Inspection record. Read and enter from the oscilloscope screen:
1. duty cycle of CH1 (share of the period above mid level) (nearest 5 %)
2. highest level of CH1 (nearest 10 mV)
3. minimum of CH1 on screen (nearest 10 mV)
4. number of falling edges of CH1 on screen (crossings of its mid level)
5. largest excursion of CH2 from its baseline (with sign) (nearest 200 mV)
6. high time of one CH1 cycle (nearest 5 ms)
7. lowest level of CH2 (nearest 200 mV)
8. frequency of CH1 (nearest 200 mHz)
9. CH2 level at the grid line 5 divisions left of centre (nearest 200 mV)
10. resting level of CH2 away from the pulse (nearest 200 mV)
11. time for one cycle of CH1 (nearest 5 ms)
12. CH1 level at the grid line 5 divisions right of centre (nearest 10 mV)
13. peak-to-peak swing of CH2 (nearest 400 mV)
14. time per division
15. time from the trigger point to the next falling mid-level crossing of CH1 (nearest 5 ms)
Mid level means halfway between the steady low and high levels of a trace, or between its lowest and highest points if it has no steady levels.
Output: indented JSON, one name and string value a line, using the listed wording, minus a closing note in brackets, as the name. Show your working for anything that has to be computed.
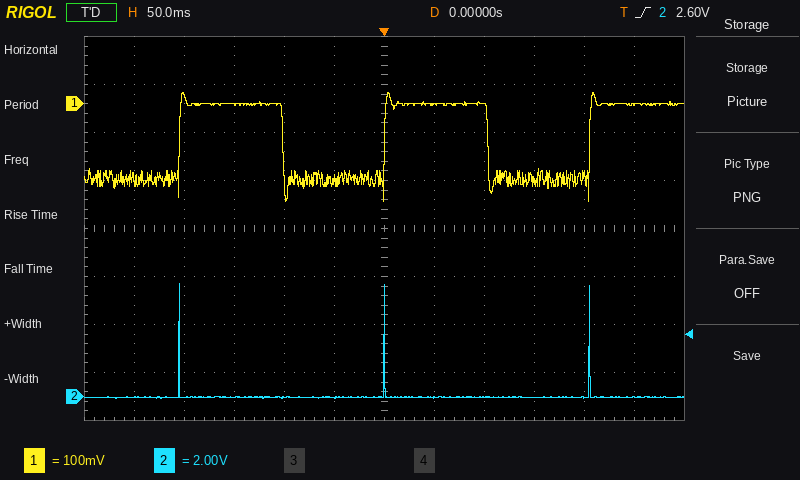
{
  "duty cycle of CH1 (share of the period above mid level)": "105 ms / 205 ms ≈ 51.2 %, so 50 % to the nearest 5 %",
  "highest level of CH1": "20 mV",
  "minimum of CH1 on screen": "-200 mV",
  "number of falling edges of CH1 on screen": "2",
  "largest excursion of CH2 from its baseline (with sign)": "+4.8 V",
  "high time of one CH1 cycle": "105 ms",
  "lowest level of CH2": "0.0 V",
  "frequency of CH1": "1 / 205 ms ≈ 4.88 Hz, so 4.8 Hz to the nearest 200 mHz",
  "CH2 level at the grid line 5 divisions left of centre": "0.0 V",
  "resting level of CH2 away from the pulse": "0.0 V",
  "time for one cycle of CH1": "205 ms",
  "CH1 level at the grid line 5 divisions right of centre": "0 mV",
  "peak-to-peak swing of CH2": "4.8 V",
  "time per division": "50 ms",
  "time from the trigger point to the next falling mid-level crossing of CH1": "105 ms"
}
